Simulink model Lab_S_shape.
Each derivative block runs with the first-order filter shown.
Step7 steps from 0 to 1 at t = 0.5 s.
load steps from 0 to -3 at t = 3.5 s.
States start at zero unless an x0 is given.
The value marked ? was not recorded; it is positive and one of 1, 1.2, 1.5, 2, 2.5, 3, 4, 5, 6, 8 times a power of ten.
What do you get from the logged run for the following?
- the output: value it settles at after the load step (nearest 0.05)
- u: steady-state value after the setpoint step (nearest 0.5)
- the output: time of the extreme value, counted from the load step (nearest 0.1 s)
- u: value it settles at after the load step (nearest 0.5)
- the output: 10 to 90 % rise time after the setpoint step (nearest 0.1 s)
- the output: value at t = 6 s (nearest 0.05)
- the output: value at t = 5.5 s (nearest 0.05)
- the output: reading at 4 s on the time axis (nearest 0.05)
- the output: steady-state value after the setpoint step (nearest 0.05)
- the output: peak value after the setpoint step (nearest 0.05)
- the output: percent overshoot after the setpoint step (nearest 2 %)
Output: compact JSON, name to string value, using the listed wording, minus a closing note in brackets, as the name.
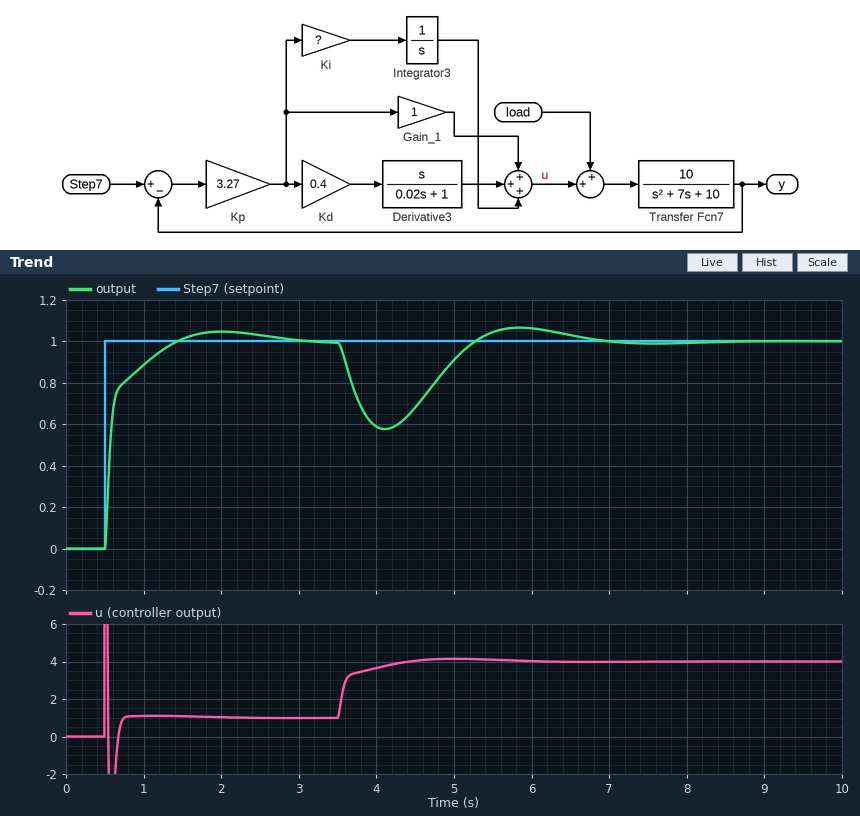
{"the output: value it settles at after the load step": "1.00", "u: steady-state value after the setpoint step": "1.0", "the output: time of the extreme value, counted from the load step": "0.6 s", "u: value it settles at after the load step": "4.0", "the output: 10 to 90 % rise time after the setpoint step": "0.5 s", "the output: value at t = 6 s": "1.05", "the output: value at t = 5.5 s": "1.05", "the output: reading at 4 s on the time axis": "0.60", "the output: steady-state value after the setpoint step": "1.00", "the output: peak value after the setpoint step": "1.05", "the output: percent overshoot after the setpoint step": "4 %"}
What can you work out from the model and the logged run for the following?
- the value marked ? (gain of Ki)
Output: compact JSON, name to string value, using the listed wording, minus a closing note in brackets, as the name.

{"the value marked ?": "2.5"}
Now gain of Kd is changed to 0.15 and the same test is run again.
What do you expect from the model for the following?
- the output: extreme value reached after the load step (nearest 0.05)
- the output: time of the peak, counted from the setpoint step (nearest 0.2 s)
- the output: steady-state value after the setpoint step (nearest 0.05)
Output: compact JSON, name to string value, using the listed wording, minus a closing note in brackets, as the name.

{"the output: extreme value reached after the load step": "0.50", "the output: time of the peak, counted from the setpoint step": "0.8 s", "the output: steady-state value after the setpoint step": "1.00"}
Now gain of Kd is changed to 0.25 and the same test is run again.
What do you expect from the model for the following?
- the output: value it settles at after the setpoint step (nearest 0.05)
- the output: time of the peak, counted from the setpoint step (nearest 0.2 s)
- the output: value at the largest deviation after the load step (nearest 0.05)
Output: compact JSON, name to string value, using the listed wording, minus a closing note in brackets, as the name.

{"the output: value it settles at after the setpoint step": "1.00", "the output: time of the peak, counted from the setpoint step": "1.2 s", "the output: value at the largest deviation after the load step": "0.55"}
